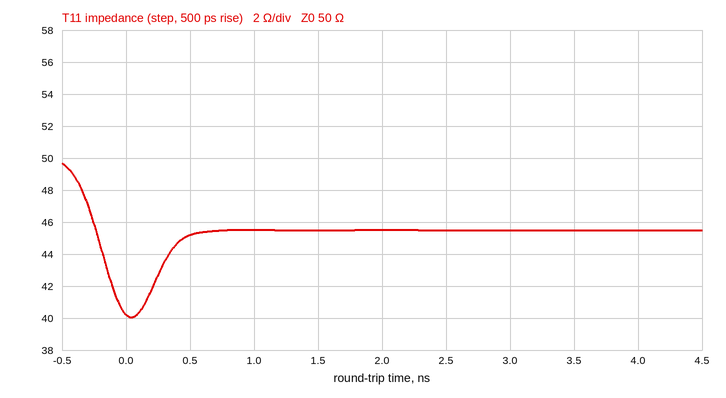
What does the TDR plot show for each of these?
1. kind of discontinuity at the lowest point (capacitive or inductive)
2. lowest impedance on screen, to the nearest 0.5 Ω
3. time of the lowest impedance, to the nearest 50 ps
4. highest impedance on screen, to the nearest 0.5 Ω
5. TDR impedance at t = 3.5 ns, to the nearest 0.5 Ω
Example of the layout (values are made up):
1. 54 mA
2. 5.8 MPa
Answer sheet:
1. capacitive
2. 40.0 Ω
3. 50 ps
4. 49.5 Ω
5. 45.5 Ω
